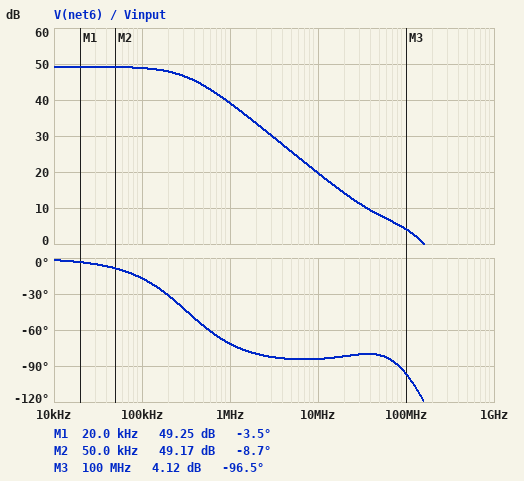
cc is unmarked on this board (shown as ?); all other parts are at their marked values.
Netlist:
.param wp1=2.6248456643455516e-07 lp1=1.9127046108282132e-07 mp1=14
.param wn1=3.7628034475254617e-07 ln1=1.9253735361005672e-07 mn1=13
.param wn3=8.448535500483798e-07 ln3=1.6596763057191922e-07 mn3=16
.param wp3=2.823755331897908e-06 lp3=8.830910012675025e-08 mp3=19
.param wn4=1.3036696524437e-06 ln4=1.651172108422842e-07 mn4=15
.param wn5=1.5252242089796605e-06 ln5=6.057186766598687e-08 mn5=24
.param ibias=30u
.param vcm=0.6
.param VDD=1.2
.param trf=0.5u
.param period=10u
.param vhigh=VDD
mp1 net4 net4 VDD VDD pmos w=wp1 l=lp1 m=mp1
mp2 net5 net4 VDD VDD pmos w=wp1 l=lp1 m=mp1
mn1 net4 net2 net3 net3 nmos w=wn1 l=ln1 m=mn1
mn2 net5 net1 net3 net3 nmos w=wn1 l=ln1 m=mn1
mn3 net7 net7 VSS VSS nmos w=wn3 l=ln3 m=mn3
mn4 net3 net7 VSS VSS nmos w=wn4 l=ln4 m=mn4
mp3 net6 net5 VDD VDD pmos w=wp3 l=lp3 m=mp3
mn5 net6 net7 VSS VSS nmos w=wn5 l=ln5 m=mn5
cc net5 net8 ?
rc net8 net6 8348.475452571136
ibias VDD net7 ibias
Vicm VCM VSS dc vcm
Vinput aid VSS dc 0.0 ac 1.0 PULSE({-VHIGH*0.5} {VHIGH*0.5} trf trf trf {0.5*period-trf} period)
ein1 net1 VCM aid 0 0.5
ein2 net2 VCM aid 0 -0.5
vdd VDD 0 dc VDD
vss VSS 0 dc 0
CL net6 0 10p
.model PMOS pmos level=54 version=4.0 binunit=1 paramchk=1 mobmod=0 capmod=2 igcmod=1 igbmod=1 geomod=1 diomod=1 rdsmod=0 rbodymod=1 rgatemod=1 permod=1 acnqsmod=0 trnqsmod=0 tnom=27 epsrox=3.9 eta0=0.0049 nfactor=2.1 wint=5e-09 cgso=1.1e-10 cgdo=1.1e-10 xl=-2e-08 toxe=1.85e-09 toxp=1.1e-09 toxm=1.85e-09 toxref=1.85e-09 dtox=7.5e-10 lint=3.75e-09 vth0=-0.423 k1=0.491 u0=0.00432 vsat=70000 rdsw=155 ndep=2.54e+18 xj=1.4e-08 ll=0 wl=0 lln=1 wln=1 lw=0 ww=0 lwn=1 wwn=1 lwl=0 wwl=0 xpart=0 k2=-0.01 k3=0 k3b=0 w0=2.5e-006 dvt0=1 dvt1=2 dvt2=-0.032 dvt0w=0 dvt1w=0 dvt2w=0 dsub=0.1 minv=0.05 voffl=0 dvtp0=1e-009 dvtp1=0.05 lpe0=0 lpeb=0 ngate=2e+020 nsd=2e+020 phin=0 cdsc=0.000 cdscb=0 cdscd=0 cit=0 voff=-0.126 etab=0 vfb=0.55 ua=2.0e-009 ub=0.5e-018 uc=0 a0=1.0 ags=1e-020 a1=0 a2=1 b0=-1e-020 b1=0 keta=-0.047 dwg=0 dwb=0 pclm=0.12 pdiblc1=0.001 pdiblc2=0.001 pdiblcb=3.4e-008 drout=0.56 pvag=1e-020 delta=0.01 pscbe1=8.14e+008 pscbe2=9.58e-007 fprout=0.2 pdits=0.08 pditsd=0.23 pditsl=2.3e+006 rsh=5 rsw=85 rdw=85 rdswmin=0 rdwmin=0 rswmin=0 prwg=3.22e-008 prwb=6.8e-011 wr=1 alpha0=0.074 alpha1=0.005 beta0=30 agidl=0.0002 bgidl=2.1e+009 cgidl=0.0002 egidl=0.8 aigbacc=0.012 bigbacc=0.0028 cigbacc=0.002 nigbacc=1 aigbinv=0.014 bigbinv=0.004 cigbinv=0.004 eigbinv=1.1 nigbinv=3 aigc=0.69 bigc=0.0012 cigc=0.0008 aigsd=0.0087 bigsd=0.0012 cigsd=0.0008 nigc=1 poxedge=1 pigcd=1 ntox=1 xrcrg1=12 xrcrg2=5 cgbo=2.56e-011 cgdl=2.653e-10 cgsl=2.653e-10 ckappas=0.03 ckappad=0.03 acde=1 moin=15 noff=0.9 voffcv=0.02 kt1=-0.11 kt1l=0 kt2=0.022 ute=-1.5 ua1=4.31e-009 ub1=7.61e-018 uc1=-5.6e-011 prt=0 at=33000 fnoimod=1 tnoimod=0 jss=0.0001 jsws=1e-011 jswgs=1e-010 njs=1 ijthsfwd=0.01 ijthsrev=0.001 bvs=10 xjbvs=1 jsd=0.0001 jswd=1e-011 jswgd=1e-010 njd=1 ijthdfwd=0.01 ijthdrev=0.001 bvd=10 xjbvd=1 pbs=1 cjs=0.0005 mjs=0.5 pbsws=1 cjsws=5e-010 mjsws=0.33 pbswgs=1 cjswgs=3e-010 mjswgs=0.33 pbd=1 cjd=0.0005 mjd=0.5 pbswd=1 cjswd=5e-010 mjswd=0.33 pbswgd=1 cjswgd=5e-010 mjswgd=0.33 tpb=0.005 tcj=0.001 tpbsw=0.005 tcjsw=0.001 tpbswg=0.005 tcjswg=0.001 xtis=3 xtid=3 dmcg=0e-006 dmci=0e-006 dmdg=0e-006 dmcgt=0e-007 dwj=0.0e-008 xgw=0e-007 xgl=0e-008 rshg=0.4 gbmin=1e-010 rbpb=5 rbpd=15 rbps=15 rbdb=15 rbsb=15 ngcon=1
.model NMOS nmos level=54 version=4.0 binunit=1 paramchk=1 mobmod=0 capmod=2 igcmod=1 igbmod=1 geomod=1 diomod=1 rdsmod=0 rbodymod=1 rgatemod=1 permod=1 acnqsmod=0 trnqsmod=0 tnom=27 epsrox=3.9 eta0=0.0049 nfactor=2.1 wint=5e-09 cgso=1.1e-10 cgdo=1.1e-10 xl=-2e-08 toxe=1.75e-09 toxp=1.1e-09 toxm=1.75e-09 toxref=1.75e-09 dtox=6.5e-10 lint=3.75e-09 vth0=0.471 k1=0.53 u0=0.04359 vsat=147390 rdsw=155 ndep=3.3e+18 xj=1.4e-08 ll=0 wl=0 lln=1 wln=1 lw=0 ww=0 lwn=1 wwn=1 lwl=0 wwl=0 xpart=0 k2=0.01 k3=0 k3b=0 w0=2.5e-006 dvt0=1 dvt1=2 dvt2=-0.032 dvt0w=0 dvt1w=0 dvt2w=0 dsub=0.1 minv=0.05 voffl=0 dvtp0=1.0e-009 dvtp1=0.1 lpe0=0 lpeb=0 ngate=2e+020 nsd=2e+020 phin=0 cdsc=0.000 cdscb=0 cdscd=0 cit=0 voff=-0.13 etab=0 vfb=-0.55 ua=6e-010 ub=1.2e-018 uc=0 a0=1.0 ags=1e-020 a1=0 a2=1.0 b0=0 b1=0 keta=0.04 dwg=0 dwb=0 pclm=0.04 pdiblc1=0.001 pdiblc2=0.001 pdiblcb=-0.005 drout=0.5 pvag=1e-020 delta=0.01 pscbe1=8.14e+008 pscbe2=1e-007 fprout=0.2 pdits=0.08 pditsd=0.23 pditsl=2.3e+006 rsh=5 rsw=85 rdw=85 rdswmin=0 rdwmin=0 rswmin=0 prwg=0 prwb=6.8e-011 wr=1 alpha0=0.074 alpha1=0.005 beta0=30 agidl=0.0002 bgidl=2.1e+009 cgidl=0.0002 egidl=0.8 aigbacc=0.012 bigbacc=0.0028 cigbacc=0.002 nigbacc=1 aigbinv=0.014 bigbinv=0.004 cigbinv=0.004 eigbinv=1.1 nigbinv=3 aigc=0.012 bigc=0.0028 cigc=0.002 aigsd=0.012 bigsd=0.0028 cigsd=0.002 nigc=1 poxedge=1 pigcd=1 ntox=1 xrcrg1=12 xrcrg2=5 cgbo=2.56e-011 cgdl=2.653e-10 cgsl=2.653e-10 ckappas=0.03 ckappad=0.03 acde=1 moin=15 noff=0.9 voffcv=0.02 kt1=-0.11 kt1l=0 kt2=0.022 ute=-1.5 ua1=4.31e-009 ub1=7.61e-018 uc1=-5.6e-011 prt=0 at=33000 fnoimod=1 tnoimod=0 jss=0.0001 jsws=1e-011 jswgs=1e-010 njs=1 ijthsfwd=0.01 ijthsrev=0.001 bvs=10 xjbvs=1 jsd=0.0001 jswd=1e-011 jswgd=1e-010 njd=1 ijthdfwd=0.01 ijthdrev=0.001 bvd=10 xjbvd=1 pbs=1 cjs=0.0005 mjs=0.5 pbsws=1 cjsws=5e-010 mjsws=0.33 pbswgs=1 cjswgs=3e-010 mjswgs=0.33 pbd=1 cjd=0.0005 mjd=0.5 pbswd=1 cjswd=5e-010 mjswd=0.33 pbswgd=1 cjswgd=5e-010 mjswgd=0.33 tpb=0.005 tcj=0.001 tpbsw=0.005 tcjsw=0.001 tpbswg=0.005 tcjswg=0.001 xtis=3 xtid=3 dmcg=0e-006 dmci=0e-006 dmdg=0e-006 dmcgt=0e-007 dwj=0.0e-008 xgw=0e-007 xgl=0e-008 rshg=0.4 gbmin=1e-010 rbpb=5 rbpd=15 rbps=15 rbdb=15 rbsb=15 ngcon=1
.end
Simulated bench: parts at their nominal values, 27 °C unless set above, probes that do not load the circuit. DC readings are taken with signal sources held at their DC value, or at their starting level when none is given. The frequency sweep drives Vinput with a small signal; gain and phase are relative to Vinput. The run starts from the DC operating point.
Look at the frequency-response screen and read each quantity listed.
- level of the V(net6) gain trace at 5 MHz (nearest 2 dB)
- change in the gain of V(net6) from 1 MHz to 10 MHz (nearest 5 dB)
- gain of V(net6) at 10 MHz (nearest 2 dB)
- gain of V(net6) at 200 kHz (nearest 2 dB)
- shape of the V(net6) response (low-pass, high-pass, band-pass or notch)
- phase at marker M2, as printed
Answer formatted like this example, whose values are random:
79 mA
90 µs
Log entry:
26 dB
-20 dB
20 dB
48 dB
low-pass
-8.7 deg
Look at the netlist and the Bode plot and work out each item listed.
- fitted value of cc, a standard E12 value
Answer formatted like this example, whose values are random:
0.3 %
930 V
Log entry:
390 fF
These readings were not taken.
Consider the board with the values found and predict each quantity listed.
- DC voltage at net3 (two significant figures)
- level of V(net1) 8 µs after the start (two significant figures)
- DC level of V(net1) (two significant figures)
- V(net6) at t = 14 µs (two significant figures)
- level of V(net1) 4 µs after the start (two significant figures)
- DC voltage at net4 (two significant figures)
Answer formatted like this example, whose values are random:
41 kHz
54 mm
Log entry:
140 mV
300 mV
600 mV
1.2 V
900 mV
570 mV
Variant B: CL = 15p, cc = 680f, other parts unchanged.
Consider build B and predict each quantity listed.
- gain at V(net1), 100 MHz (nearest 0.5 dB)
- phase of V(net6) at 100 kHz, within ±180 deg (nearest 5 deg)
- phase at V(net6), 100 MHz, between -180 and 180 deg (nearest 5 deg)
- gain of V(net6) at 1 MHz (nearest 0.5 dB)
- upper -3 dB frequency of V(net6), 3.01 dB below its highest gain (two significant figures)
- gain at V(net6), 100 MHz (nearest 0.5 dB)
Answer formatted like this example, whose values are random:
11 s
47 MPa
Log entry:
-6.0 dB
-25 deg
-100 deg
35.0 dB
200 kHz
2.0 dB
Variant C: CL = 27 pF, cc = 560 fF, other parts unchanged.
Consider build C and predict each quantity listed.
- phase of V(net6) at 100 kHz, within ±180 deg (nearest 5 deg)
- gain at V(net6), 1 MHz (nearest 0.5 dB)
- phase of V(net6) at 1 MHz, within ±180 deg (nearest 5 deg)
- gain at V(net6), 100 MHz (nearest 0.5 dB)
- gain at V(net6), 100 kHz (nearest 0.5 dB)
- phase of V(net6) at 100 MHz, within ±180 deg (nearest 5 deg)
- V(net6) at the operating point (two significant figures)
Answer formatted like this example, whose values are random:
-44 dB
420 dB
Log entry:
-25 deg
36.5 dB
-75 deg
-2.5 dB
48.5 dB
-120 deg
1.0 V
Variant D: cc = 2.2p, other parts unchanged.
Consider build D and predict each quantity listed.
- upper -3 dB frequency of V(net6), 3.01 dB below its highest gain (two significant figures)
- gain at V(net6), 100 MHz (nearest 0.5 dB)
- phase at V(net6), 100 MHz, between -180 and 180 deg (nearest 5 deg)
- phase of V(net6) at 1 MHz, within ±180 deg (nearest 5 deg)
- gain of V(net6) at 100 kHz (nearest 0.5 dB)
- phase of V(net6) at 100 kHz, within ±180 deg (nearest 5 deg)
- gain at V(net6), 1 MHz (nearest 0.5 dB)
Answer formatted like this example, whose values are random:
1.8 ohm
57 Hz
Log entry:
65 kHz
4.5 dB
-75 deg
-80 deg
44.0 dB
-55 deg
25.5 dB
